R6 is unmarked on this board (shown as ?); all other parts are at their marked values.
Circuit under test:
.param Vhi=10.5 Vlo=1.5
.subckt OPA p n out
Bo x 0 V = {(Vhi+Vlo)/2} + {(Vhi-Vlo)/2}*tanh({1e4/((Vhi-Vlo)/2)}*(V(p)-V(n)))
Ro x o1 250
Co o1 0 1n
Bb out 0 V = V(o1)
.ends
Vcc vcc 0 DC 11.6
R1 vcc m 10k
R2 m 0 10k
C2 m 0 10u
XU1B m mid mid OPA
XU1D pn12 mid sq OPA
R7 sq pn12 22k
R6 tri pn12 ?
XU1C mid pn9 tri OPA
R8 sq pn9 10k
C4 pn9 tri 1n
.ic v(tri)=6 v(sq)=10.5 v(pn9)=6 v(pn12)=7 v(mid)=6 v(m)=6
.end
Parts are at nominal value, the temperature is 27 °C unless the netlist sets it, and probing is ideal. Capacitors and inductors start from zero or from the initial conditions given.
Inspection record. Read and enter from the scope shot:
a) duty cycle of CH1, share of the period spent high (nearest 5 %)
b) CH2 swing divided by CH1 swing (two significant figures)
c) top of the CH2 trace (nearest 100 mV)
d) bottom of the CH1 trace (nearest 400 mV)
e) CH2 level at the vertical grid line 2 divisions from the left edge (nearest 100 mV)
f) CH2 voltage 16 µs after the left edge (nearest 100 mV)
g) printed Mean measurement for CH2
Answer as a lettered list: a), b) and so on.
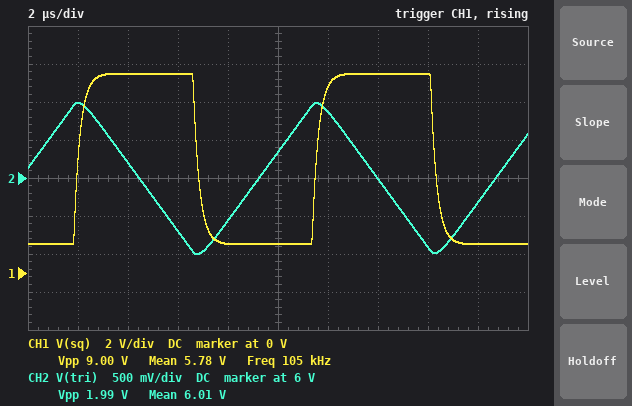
a) 50 %
b) 0.22
c) 7.0 V
d) 1.6 V
e) 6.2 V
f) 5.1 V
g) 6.01 V
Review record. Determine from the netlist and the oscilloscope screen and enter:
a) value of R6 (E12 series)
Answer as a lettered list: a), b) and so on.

a) 4.7 kΩ
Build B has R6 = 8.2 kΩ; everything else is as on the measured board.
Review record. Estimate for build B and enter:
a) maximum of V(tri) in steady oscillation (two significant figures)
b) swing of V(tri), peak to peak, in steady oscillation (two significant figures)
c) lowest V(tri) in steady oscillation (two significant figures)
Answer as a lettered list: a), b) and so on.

a) 7.7 V
b) 3.4 V
c) 4.3 V
